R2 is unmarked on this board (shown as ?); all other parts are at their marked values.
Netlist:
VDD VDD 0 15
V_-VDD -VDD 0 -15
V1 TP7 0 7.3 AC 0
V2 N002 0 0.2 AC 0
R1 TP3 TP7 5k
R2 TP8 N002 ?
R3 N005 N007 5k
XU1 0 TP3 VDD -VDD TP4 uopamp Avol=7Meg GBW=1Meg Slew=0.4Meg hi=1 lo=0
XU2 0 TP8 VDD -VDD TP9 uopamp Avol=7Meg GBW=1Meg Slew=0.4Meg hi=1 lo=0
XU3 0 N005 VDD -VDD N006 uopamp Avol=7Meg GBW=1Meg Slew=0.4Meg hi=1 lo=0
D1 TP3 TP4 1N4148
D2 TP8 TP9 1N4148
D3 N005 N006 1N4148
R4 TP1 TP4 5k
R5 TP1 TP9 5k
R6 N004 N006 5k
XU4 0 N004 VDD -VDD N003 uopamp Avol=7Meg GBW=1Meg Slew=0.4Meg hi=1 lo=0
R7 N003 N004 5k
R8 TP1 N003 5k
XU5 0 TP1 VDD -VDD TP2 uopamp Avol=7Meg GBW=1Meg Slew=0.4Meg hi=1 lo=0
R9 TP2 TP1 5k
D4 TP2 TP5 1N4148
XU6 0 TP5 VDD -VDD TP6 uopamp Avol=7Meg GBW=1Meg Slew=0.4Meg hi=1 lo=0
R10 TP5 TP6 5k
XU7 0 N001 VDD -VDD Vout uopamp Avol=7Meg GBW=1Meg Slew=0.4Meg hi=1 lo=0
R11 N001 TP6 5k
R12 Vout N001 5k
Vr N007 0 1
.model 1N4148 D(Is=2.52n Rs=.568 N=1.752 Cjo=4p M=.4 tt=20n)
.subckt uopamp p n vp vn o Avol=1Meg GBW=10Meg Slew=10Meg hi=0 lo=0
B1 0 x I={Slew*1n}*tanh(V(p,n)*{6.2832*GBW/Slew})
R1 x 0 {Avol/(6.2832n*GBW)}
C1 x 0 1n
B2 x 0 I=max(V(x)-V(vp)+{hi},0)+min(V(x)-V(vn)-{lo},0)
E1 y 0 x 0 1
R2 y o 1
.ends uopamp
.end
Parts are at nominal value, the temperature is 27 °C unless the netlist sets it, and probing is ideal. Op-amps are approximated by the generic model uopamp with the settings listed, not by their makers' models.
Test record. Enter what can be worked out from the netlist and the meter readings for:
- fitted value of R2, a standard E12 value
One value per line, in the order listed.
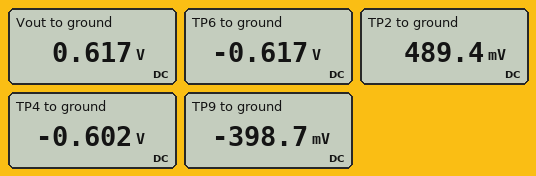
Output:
12 kΩ
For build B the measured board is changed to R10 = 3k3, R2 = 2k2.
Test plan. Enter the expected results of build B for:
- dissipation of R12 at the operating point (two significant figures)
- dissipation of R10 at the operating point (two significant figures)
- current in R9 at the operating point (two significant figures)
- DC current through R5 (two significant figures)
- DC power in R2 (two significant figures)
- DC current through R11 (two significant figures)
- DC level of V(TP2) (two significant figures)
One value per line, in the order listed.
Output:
980 µW
1.5 mW
110 µA
95 µA
18 µW
440 µA
570 mV
